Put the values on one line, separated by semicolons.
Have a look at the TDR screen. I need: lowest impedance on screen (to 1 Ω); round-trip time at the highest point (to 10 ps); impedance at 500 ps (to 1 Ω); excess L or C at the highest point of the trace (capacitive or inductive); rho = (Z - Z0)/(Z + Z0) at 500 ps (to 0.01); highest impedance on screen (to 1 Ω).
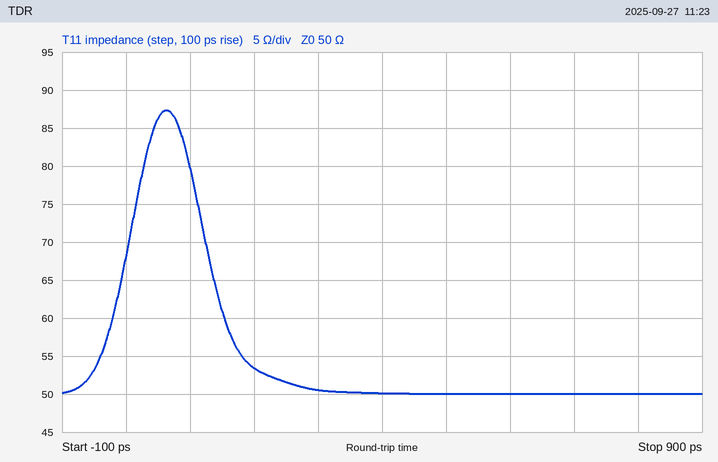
50 Ω; 60 ps; 50 Ω; inductive; 0.00; 87 Ω
